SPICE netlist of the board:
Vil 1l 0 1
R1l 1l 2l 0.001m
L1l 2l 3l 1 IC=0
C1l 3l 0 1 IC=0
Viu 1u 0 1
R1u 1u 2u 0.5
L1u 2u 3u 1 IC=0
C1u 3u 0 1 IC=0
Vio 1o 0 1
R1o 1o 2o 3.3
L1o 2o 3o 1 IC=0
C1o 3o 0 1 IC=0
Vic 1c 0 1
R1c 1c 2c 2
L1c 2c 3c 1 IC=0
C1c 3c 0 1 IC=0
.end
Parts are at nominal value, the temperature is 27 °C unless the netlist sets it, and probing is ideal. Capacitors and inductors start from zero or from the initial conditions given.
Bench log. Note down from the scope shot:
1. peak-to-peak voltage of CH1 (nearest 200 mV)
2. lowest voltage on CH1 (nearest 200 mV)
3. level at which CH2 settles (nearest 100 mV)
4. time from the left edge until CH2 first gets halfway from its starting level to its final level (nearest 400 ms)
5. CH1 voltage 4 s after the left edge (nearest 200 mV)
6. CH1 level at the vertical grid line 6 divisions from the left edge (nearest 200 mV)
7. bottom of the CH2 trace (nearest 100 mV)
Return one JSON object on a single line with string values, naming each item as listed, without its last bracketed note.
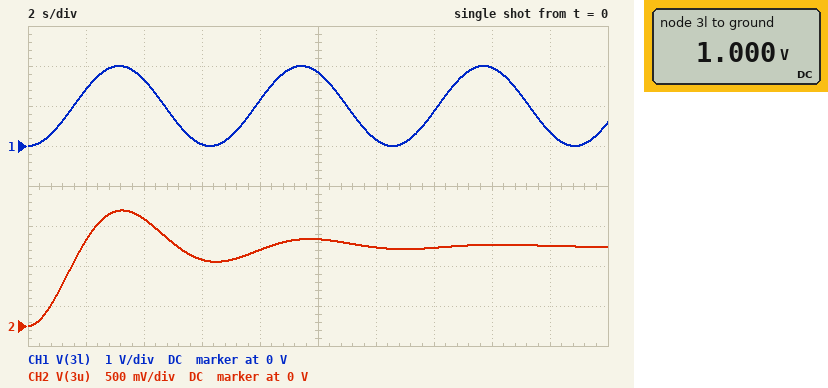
{"peak-to-peak voltage of CH1": "2.0 V", "lowest voltage on CH1": "0 V", "level at which CH2 settles": "1.0 V", "time from the left edge until CH2 first gets halfway from its starting level to its final level": "1.2 s", "CH1 voltage 4 s after the left edge": "1.6 V", "CH1 level at the vertical grid line 6 divisions from the left edge": "200 mV", "bottom of the CH2 trace": "0 V"}
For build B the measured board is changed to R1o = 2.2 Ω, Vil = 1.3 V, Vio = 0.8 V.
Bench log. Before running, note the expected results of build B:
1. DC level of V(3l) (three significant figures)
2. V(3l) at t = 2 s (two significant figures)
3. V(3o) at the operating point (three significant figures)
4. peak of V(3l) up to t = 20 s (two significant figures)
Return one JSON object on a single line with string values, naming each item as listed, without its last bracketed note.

{"DC level of V(3l)": "1.30 V", "V(3l) at t = 2 s": "1.8 V", "V(3o) at the operating point": "800 mV", "peak of V(3l) up to t = 20 s": "2.6 V"}
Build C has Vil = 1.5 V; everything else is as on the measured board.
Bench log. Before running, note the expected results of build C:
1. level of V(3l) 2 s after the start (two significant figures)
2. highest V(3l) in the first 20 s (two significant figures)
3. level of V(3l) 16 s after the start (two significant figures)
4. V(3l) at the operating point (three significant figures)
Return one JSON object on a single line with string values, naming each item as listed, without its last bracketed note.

{"level of V(3l) 2 s after the start": "2.1 V", "highest V(3l) in the first 20 s": "3.0 V", "level of V(3l) 16 s after the start": "2.9 V", "V(3l) at the operating point": "1.50 V"}
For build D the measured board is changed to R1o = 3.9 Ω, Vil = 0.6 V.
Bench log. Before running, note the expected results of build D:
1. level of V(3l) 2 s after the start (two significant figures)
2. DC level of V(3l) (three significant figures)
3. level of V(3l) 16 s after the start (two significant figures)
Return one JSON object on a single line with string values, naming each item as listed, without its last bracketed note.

{"level of V(3l) 2 s after the start": "850 mV", "DC level of V(3l)": "600 mV", "level of V(3l) 16 s after the start": "1.2 V"}
